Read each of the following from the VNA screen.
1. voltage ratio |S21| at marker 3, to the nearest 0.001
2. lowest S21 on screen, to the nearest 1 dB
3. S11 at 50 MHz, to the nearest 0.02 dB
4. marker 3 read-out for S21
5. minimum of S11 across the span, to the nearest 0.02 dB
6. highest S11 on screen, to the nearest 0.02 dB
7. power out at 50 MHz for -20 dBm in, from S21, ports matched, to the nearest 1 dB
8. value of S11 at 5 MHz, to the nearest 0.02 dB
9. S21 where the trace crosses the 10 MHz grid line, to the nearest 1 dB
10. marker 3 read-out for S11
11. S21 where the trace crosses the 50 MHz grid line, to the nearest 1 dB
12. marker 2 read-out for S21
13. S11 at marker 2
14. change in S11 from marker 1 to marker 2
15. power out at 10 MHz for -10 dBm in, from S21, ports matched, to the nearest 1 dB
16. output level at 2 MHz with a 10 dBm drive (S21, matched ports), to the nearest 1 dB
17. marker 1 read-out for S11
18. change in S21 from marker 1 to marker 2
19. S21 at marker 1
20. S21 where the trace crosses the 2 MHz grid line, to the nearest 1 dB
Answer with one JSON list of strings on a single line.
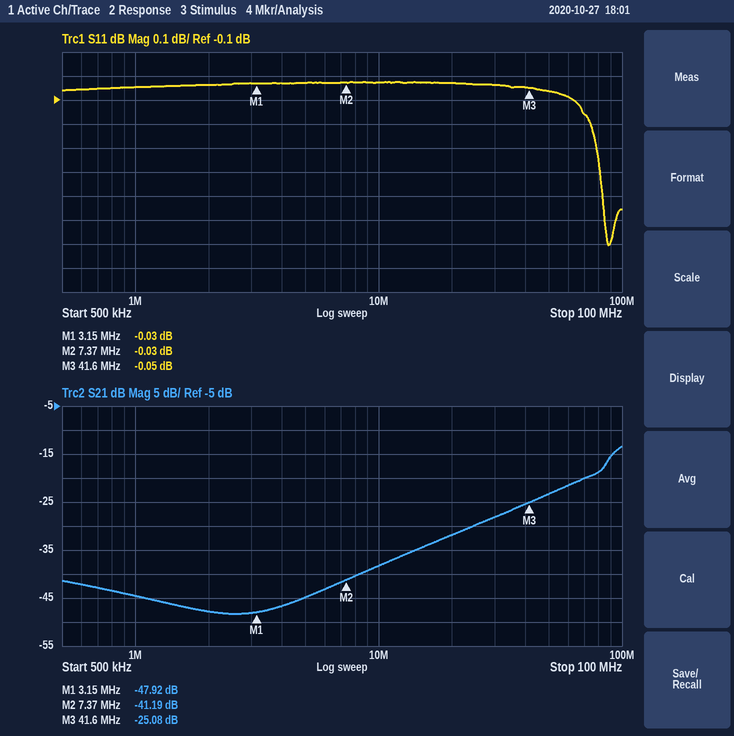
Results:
["0.056", "-48 dB", "-0.06 dB", "-25.08 dB", "-0.70 dB", "-0.02 dB", "-43 dBm", "-0.02 dB", "-38 dB", "-0.05 dB", "-23 dB", "-41.19 dB", "-0.03 dB", "0.00 dB", "-48 dBm", "-38 dBm", "-0.03 dB", "6.73 dB", "-47.92 dB", "-48 dB"]
